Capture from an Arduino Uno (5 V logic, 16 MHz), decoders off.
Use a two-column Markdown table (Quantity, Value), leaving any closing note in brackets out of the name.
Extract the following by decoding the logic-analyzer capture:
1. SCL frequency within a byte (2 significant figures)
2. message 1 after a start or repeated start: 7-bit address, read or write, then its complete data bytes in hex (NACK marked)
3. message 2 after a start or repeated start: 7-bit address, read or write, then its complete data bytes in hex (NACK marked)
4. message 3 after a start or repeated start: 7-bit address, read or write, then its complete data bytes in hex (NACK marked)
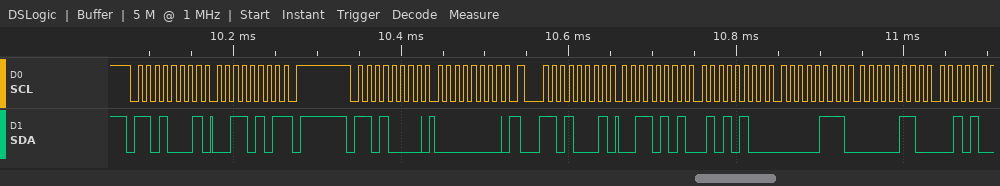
| Quantity | Value |
|---|---|
| SCL frequency within a byte | 100 kHz |
| message 1 after a start or repeated start: 7-bit address, read or write, then its complete data bytes in hex | 0x68 read: 35 NACK |
| message 2 after a start or repeated start: 7-bit address, read or write, then its complete data bytes in hex | 0x68 write: 00 |
| message 3 after a start or repeated start: 7-bit address, read or write, then its complete data bytes in hex | 0x68 read: 35 54 07 06 |
